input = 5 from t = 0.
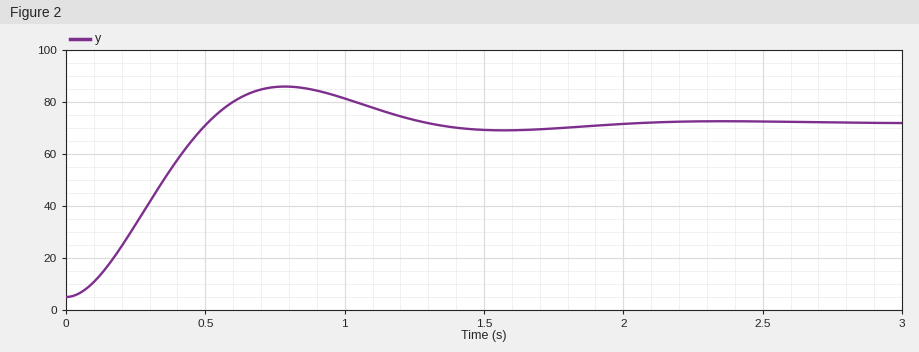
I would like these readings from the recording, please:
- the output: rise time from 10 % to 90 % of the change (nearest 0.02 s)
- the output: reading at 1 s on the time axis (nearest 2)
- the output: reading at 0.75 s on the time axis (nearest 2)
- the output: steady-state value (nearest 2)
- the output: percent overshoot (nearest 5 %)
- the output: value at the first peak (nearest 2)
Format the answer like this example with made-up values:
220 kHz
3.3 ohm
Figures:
0.34 s
82
86
72
20 %
86
